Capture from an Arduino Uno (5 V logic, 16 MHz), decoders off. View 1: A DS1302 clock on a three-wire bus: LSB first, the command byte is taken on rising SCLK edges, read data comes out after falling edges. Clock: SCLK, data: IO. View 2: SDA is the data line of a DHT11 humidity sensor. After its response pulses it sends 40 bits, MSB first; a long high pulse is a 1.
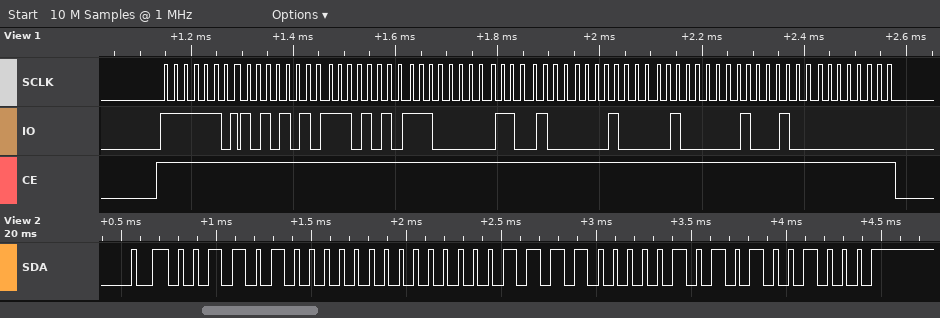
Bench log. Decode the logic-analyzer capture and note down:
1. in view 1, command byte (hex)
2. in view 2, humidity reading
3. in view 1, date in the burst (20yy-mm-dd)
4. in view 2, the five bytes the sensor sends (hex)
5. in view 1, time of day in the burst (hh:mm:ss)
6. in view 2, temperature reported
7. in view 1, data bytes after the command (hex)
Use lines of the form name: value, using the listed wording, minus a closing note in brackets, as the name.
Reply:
in view 1, command byte: 0xBF
in view 2, humidity reading: 52 %
in view 1, date in the burst: 2022-10-26
in view 2, the five bytes the sensor sends: 34 00 0F 05 48
in view 1, time of day in the burst: 07:57:55
in view 2, temperature reported: 15.5 °C
in view 1, data bytes after the command: 55 57 07 26 10 04 22 00
